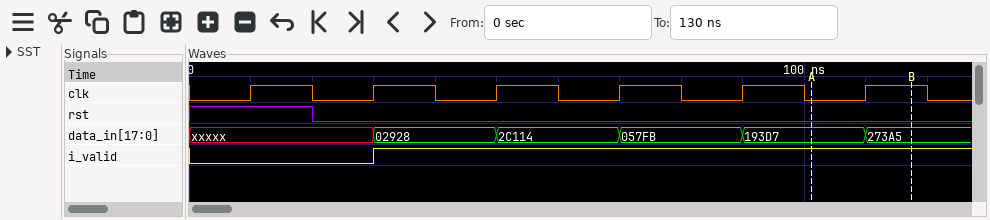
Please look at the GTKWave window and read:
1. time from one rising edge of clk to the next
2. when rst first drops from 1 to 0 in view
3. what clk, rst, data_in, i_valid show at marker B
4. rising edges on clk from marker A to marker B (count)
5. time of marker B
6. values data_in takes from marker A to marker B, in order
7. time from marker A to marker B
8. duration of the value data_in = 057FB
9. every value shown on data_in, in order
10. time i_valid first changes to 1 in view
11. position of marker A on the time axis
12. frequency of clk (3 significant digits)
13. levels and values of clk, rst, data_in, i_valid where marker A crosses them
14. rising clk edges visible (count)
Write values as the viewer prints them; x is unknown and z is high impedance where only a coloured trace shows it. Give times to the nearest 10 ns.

20 ns
20 ns
clk=1, rst=0, data_in=273A5, i_valid=1
1
120 ns
193D7, 273A5
20 ns
20 ns
xxxxx, 02928, 2C114, 057FB, 193D7, 273A5
30 ns
100 ns
50.0 MHz
clk=0, rst=0, data_in=193D7, i_valid=1
6
